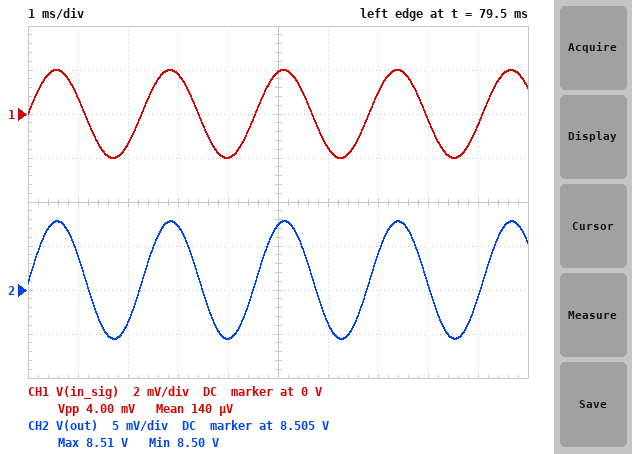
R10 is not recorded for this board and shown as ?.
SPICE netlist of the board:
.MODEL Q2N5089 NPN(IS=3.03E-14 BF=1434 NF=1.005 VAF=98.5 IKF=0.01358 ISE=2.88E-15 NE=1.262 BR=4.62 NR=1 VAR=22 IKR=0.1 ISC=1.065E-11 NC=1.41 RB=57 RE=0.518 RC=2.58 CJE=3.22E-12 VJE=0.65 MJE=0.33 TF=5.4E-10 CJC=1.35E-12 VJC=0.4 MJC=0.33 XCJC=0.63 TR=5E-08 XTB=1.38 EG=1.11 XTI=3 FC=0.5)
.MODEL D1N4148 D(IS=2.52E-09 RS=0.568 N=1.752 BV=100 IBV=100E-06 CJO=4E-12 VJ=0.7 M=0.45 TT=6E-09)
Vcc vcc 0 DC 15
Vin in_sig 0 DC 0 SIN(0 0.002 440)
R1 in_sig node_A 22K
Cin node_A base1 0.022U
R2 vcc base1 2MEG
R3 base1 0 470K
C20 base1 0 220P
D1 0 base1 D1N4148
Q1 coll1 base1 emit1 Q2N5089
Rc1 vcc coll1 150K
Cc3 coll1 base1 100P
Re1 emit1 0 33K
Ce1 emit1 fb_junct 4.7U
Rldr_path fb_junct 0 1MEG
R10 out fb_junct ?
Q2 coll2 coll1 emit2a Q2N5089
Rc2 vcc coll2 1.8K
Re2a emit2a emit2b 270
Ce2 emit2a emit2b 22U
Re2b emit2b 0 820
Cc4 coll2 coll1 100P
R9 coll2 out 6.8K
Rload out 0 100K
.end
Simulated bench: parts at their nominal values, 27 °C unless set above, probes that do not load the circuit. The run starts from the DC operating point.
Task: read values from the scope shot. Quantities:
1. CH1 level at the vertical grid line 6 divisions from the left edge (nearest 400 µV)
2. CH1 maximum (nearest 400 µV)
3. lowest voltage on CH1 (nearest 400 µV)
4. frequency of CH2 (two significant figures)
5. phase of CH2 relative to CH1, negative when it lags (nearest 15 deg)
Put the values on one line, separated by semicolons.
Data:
-1.6 mV; 2.0 mV; -2.0 mV; 440 Hz; 0 deg
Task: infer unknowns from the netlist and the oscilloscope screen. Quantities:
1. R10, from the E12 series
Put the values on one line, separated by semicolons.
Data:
180 kΩ
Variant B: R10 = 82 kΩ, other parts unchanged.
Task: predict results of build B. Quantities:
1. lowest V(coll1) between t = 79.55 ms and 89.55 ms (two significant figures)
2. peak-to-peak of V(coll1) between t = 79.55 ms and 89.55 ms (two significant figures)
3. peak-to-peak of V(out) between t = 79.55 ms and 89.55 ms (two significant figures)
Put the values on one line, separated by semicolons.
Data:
4.1 V; 5.1 mV; 9.5 mV
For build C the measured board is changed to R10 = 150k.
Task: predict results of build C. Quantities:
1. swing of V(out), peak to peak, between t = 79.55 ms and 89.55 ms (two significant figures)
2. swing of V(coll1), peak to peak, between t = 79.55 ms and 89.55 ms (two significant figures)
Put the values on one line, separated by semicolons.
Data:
12 mV; 6.5 mV
